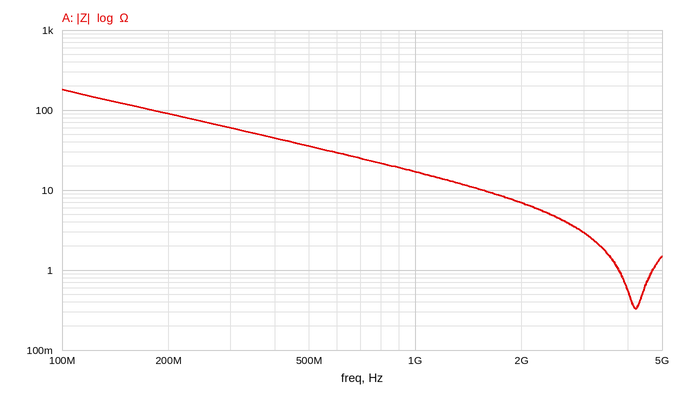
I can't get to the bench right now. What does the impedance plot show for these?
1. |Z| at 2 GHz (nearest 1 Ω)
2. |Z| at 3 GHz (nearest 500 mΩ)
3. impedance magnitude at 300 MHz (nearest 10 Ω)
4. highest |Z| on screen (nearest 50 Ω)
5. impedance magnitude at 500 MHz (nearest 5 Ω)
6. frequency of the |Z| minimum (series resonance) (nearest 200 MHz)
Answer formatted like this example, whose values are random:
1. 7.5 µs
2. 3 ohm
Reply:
1. 7 Ω
2. 3.0 Ω
3. 60 Ω
4. 200 Ω
5. 35 Ω
6. 4.2 GHz
